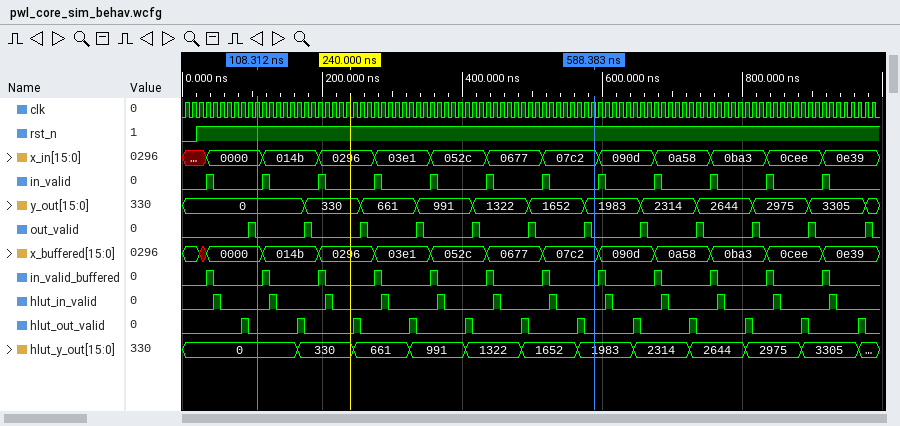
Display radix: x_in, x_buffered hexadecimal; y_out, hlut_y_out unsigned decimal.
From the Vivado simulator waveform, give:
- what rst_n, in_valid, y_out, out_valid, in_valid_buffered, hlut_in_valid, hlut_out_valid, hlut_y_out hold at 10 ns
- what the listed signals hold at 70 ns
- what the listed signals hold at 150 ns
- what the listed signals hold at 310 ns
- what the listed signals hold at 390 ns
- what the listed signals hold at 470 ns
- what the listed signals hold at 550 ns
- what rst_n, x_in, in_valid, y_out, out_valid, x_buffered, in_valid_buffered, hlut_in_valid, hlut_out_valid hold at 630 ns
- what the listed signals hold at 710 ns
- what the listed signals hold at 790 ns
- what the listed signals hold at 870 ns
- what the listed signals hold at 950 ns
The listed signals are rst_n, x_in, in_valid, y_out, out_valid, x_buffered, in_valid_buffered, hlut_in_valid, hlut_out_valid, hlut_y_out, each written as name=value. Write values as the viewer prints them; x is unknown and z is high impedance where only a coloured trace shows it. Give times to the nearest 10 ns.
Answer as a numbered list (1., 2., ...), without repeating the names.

1. rst_n=0, in_valid=0, y_out=0, out_valid=0, in_valid_buffered=0, hlut_in_valid=0, hlut_out_valid=0, hlut_y_out=0
2. rst_n=1, x_in=0000, in_valid=0, y_out=0, out_valid=0, x_buffered=0000, in_valid_buffered=0, hlut_in_valid=0, hlut_out_valid=0, hlut_y_out=0
3. rst_n=1, x_in=014b, in_valid=0, y_out=0, out_valid=0, x_buffered=014b, in_valid_buffered=0, hlut_in_valid=0, hlut_out_valid=0, hlut_y_out=0
4. rst_n=1, x_in=03e1, in_valid=0, y_out=661, out_valid=0, x_buffered=03e1, in_valid_buffered=0, hlut_in_valid=0, hlut_out_valid=0, hlut_y_out=661
5. rst_n=1, x_in=052c, in_valid=0, y_out=991, out_valid=0, x_buffered=052c, in_valid_buffered=0, hlut_in_valid=0, hlut_out_valid=0, hlut_y_out=991
6. rst_n=1, x_in=0677, in_valid=0, y_out=1322, out_valid=0, x_buffered=0677, in_valid_buffered=0, hlut_in_valid=0, hlut_out_valid=0, hlut_y_out=1322
7. rst_n=1, x_in=07c2, in_valid=0, y_out=1652, out_valid=0, x_buffered=07c2, in_valid_buffered=0, hlut_in_valid=0, hlut_out_valid=0, hlut_y_out=1652
8. rst_n=1, x_in=090d, in_valid=0, y_out=1983, out_valid=0, x_buffered=090d, in_valid_buffered=0, hlut_in_valid=0, hlut_out_valid=0
9. rst_n=1, x_in=0a58, in_valid=0, y_out=2314, out_valid=0, x_buffered=0a58, in_valid_buffered=0, hlut_in_valid=0, hlut_out_valid=0, hlut_y_out=2314
10. rst_n=1, x_in=0ba3, in_valid=0, y_out=2644, out_valid=0, x_buffered=0ba3, in_valid_buffered=0, hlut_in_valid=0, hlut_out_valid=0, hlut_y_out=2644
11. rst_n=1, x_in=0cee, in_valid=0, y_out=2975, out_valid=0, x_buffered=0cee, in_valid_buffered=0, hlut_in_valid=0, hlut_out_valid=0, hlut_y_out=2975
12. rst_n=1, x_in=0e39, in_valid=0, y_out=3305, out_valid=0, x_buffered=0e39, in_valid_buffered=0, hlut_in_valid=0, hlut_out_valid=0, hlut_y_out=3305
